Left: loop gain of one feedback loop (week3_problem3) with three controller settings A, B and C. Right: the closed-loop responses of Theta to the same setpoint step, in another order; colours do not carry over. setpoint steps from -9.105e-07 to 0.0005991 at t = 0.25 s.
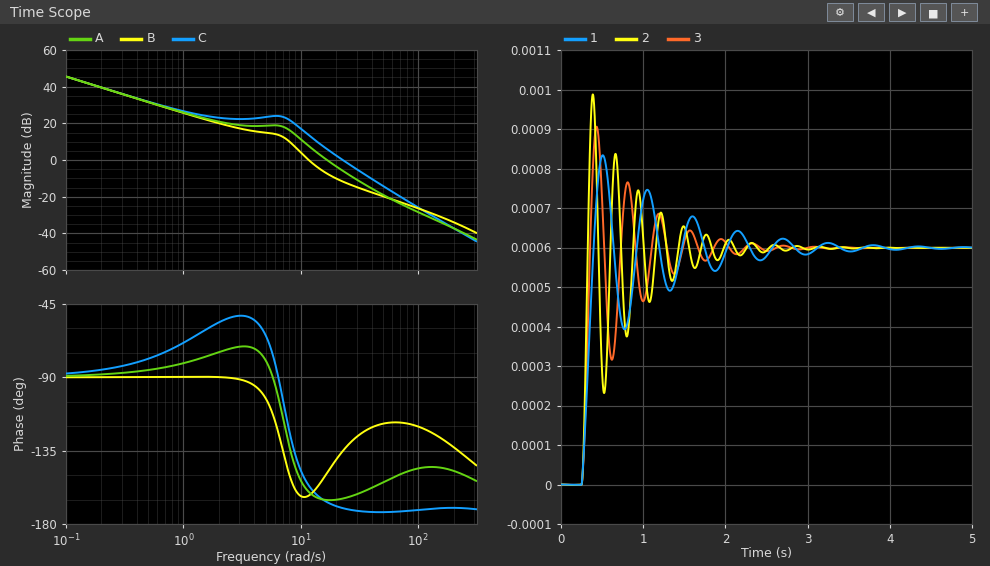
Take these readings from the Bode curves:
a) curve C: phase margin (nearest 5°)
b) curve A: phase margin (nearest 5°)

10°
15°
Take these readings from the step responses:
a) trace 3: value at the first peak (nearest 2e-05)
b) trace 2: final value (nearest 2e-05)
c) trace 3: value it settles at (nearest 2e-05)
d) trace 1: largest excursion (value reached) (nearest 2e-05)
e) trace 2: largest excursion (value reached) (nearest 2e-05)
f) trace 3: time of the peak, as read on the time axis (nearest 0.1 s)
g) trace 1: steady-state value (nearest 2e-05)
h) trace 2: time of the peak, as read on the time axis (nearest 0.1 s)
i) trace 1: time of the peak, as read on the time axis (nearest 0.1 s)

0.00090
0.00060
0.00060
0.00084
0.00098
0.4 s
0.00060
0.4 s
0.5 s
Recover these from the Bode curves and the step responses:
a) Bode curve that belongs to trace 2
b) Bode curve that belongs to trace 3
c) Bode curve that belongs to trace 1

C
A
B
